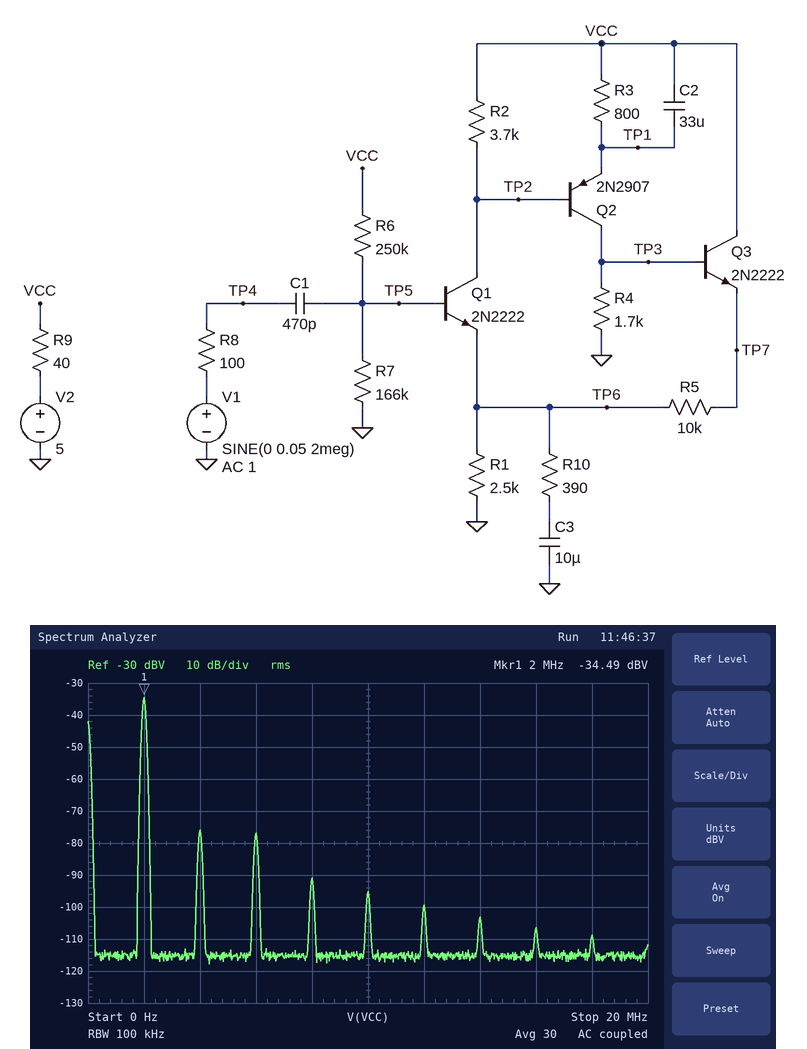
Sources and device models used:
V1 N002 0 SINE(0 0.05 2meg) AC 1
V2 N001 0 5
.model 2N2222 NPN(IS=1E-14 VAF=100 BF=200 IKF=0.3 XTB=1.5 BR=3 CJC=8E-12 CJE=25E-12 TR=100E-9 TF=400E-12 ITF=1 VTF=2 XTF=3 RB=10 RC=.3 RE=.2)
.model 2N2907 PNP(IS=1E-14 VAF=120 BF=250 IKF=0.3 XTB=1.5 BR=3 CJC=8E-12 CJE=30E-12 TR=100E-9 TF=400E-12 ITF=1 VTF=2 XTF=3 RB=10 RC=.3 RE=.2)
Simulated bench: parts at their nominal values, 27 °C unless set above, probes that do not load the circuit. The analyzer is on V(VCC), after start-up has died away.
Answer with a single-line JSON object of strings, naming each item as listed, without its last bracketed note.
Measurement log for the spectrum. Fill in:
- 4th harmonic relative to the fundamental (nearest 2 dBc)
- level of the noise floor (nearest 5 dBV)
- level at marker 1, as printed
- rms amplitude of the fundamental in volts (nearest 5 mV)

{"4th harmonic relative to the fundamental": "-56 dBc", "level of the noise floor": "-115 dBV", "level at marker 1, as printed": "-34.49 dBV", "rms amplitude of the fundamental in volts": "20 mV"}
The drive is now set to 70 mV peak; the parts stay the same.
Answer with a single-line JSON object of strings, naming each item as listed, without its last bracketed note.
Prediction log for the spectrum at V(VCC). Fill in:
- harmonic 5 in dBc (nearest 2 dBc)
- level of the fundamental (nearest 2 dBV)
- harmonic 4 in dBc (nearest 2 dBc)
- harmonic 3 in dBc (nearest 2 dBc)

{"harmonic 5 in dBc": "-56 dBc", "level of the fundamental": "-32 dBV", "harmonic 4 in dBc": "-50 dBc", "harmonic 3 in dBc": "-36 dBc"}
